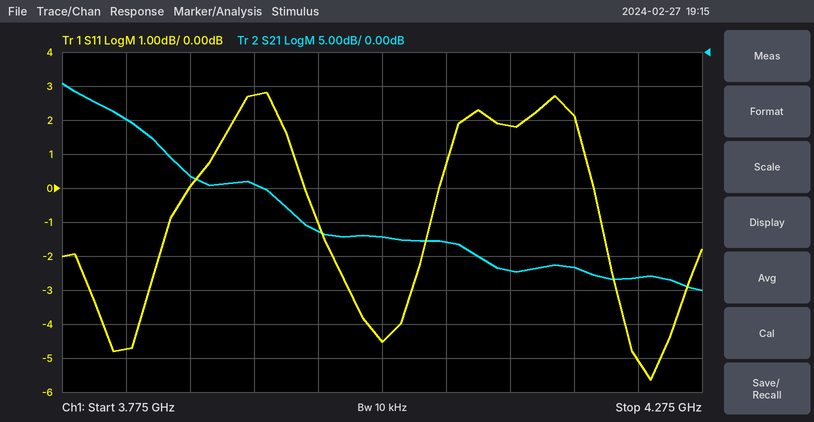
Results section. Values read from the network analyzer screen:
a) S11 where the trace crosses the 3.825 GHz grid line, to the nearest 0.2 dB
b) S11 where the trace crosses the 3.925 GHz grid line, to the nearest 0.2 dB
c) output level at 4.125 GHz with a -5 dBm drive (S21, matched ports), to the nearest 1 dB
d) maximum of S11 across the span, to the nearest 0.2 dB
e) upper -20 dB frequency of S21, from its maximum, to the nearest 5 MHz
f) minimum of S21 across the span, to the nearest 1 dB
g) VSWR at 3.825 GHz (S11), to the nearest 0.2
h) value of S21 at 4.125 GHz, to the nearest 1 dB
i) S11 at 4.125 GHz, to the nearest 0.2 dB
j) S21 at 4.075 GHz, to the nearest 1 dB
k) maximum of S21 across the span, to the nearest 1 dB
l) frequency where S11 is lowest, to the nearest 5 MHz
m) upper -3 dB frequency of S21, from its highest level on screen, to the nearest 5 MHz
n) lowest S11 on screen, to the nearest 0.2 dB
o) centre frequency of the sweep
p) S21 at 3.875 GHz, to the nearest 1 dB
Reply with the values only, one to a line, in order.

-4.8 dB
2.8 dB
-37 dBm
2.8 dB
3.960 GHz
-35 dB
3.8
-32 dB
1.8 dB
-28 dB
-5 dB
4.235 GHz
3.805 GHz
-5.6 dB
4.025 GHz
-18 dB
